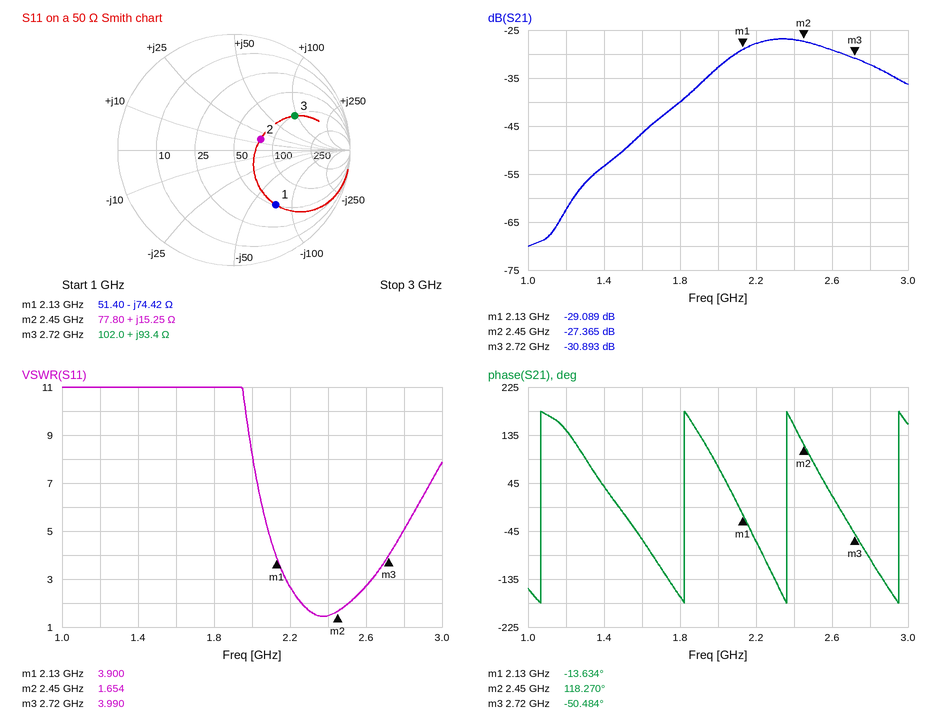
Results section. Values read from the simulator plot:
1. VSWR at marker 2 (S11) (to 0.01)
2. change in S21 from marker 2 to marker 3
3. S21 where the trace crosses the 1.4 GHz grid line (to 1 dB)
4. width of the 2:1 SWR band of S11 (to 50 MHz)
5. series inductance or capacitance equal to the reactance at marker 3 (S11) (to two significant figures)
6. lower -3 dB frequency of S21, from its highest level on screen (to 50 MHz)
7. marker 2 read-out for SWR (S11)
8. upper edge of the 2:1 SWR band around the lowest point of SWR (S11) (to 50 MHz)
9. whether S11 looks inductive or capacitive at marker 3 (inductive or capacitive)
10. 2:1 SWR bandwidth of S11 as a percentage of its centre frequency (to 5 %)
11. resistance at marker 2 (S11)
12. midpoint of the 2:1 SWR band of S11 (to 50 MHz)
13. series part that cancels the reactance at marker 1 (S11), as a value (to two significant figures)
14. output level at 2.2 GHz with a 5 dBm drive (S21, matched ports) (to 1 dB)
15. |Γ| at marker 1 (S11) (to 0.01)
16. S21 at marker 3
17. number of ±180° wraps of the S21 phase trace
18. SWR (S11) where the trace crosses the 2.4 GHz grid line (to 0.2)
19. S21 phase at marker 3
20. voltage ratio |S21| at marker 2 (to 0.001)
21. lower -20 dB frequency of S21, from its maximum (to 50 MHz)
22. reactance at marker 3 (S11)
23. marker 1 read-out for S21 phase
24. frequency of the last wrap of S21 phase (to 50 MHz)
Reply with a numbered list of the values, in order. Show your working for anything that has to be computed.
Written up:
1. 1.65
2. -30.893 − (-27.365) = -3.528 dB
3. -53 dB
4. 2.50 GHz − 2.25 GHz = 250 MHz
5. L = 93.4 Ω/(2π × 2.72 GHz) ≈ 5.5 nH
6. 2.10 GHz
7. 1.654
8. 2.50 GHz
9. inductive
10. 250 MHz / 2.375 GHz ≈ 10 %
11. 77.80 Ω
12. 2.40 GHz
13. L = 74.42 Ω/(2π × 2.13 GHz) ≈ 5.6 nH
14. 5 dBm + (-28 dB) = -23 dBm
15. 0.59
16. -30.893 dB
17. 4
18. 1.4
19. -50.484°
20. 10^(-27.365/20) ≈ 0.043
21. 1.60 GHz
22. +93.4 Ω
23. -13.634°
24. 2.95 GHz
